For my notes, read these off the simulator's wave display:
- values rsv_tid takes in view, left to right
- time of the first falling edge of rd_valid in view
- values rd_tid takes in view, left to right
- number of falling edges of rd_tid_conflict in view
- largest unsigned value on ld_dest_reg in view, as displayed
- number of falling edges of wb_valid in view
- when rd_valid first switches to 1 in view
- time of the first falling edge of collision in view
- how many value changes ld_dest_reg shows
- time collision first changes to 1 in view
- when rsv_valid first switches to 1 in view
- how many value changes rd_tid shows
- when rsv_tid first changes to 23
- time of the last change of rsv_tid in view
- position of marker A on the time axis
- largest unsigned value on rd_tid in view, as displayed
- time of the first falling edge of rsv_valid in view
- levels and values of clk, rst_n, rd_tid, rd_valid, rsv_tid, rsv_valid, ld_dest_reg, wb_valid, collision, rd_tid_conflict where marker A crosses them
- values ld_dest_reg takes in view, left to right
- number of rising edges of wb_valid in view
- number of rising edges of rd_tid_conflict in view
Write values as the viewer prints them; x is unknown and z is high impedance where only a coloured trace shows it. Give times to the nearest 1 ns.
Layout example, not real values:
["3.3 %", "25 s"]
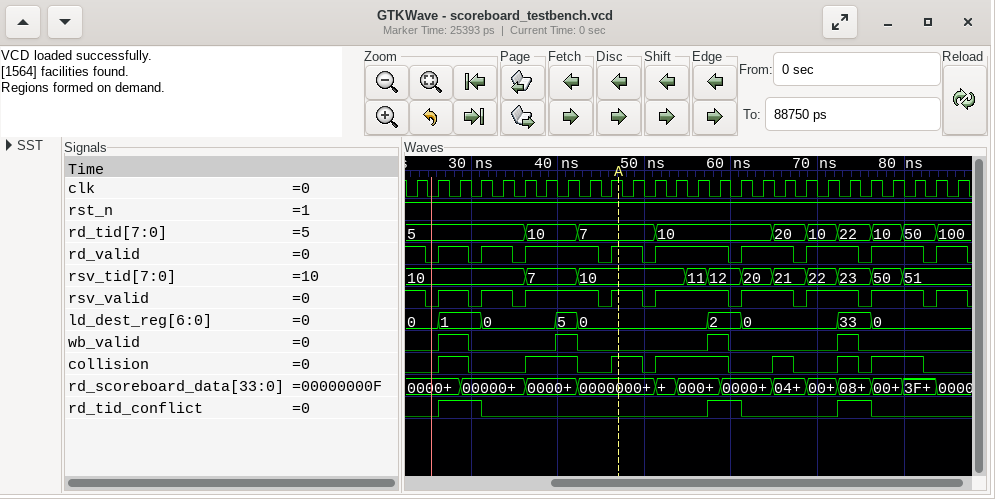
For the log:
["10, 7, 10, 11, 12, 20, 21, 22, 23, 50, 51", "25 ns", "5, 10, 7, 10, 20, 10, 22, 10, 50, 100", "3", "33", "4", "26 ns", "30 ns", "8", "26 ns", "26 ns", "9", "72 ns", "80 ns", "47 ns", "100", "25 ns", "clk=1, rst_n=1, rd_tid=7, rd_valid=1, rsv_tid=10, rsv_valid=1, ld_dest_reg=0, wb_valid=0, collision=1, rd_tid_conflict=0", "0, 1, 0, 5, 0, 2, 0, 33, 0", "4", "3"]
